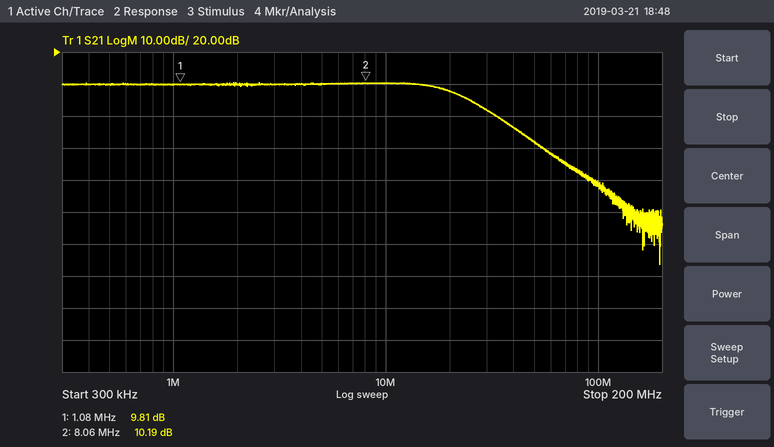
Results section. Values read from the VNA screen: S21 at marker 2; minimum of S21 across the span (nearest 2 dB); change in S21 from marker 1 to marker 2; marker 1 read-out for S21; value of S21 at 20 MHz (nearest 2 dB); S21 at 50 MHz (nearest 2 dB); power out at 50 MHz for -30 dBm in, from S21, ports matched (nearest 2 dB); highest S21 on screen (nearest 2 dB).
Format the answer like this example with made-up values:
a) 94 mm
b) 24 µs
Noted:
a) 10.19 dB
b) -46 dB
c) 0.38 dB
d) 9.81 dB
e) 8 dB
f) -8 dB
g) -38 dBm
h) 10 dB
